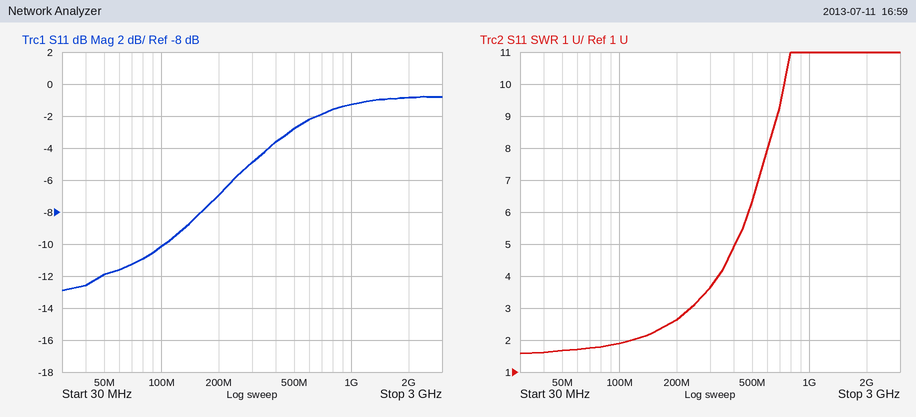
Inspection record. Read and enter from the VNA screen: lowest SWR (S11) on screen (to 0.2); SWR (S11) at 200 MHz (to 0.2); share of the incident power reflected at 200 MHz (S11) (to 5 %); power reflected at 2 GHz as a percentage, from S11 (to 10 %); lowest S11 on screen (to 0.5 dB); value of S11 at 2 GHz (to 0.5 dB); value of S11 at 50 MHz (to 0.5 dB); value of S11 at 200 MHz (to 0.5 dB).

1.6
2.6
20 %
80 %
-13.0 dB
-1.0 dB
-12.0 dB
-7.0 dB
